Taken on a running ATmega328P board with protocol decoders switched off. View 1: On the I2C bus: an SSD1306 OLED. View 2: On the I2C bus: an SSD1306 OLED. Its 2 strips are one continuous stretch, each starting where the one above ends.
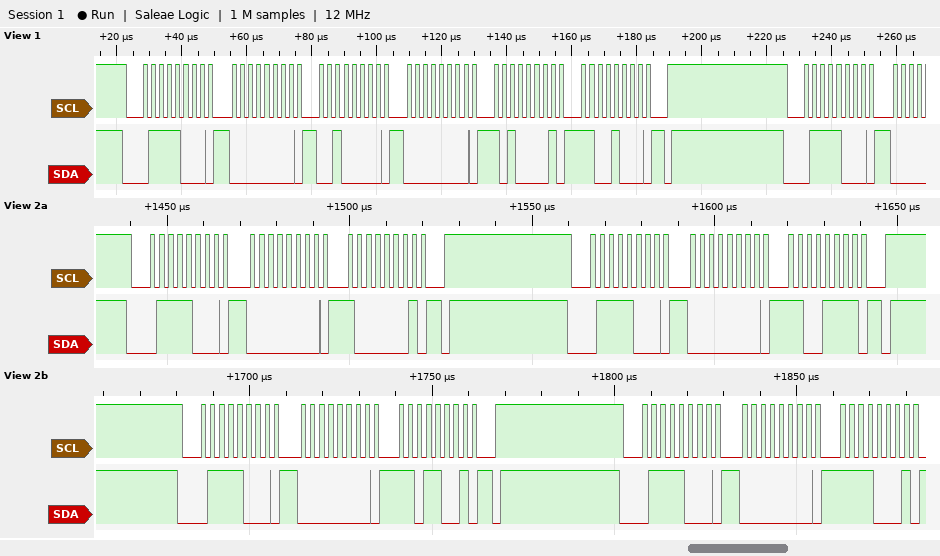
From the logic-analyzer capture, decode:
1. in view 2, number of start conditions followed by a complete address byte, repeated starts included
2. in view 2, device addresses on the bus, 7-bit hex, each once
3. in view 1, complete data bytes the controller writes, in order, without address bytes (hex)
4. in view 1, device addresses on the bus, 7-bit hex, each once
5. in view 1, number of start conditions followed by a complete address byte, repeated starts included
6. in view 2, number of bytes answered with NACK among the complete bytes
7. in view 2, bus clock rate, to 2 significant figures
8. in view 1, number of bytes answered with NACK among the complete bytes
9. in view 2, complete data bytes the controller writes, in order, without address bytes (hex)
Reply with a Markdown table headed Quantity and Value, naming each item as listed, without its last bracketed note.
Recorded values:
| Quantity | Value |
|---|---|
| in view 2, number of start conditions followed by a complete address byte, repeated starts included | 4 |
| in view 2, device addresses on the bus, 7-bit hex, each once | 0x3C |
| in view 1, complete data bytes the controller writes, in order, without address bytes | 00 20 00 A1 C8 |
| in view 1, device addresses on the bus, 7-bit hex, each once | 0x3C |
| in view 1, number of start conditions followed by a complete address byte, repeated starts included | 2 |
| in view 2, number of bytes answered with NACK among the complete bytes | 0 |
| in view 2, bus clock rate, to 2 significant figures | 400 kHz |
| in view 1, number of bytes answered with NACK among the complete bytes | 0 |
| in view 2, complete data bytes the controller writes, in order, without address bytes | 00 81 00 CF 00 D9 00 F1 |
